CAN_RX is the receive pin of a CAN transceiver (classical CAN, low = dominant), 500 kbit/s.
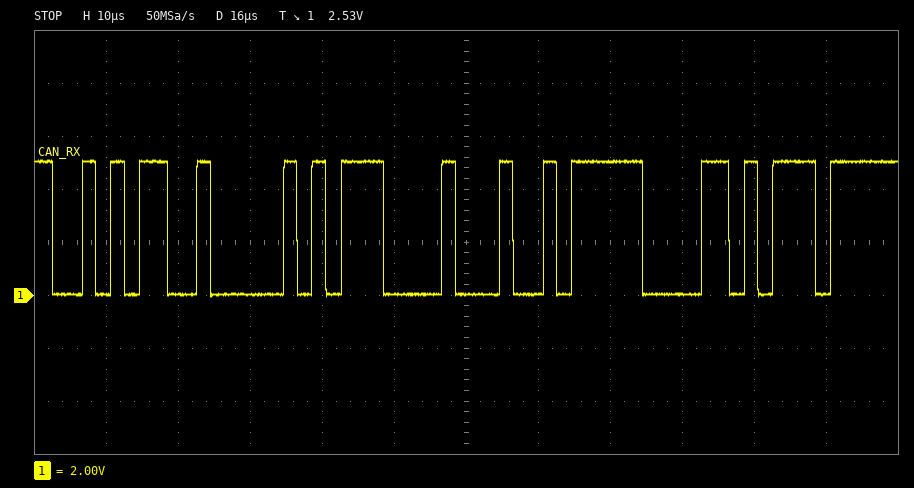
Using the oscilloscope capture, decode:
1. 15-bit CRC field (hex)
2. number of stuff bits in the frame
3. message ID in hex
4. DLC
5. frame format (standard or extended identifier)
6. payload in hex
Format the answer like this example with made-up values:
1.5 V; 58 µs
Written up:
0x7C6B; 2; 0x2B2; 2; standard; E1 12
